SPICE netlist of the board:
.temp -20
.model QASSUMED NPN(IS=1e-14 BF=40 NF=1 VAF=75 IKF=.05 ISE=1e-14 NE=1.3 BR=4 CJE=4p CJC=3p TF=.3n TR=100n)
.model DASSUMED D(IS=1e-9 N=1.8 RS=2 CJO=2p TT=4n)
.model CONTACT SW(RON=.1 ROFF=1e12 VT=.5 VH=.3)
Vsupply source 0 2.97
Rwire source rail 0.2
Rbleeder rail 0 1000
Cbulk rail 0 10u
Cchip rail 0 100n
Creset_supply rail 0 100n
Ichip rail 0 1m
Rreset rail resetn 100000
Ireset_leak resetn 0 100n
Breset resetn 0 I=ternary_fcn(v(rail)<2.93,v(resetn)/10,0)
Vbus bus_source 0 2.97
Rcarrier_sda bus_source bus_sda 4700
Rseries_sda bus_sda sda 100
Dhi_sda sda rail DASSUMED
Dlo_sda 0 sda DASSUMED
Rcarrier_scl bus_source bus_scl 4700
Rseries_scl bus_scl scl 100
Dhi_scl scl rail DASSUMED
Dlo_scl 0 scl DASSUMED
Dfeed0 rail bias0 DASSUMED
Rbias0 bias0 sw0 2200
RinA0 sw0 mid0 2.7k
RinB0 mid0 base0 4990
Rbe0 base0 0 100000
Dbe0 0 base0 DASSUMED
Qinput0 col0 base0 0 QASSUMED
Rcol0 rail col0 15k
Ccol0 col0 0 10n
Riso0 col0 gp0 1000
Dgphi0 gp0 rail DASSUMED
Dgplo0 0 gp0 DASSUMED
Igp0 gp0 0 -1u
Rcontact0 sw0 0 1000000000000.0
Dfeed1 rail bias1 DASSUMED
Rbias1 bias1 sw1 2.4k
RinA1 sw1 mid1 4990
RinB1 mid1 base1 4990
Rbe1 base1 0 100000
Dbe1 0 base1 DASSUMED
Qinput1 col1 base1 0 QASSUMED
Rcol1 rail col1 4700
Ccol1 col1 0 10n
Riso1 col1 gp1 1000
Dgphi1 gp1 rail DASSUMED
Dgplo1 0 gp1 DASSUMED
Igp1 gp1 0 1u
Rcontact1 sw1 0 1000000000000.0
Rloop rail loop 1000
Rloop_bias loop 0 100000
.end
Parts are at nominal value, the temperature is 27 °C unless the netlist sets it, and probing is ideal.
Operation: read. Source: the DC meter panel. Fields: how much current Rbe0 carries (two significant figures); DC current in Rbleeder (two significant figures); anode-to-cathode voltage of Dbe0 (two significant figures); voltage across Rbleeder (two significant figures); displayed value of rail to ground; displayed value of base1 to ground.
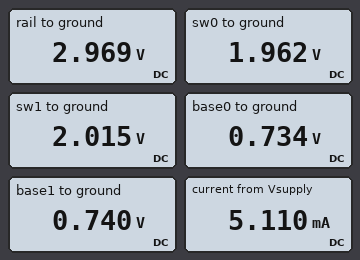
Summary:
7.3 µA
3.0 mA
-730 mV
3.0 V
2.969 V
0.740 V
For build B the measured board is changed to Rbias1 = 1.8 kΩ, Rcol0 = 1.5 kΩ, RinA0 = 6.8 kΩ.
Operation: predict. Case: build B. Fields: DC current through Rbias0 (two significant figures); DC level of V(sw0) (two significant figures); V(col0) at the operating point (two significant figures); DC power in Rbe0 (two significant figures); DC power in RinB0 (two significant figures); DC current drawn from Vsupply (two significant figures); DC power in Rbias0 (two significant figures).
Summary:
110 µA
2.1 V
56 mV
5.7 µW
63 µW
6.8 mA
28 µW
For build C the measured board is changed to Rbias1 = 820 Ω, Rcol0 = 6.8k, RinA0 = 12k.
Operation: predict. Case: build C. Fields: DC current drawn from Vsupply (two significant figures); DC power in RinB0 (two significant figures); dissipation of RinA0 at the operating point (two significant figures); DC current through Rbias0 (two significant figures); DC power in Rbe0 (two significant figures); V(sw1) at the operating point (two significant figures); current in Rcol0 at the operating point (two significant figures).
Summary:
5.3 mA
35 µW
84 µW
84 µA
5.3 µW
2.2 V
430 µA
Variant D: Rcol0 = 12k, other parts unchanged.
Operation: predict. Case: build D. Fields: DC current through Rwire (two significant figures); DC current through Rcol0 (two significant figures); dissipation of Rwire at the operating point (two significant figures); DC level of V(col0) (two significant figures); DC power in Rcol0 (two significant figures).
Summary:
5.2 mA
250 µA
5.3 µW
12 mV
730 µW
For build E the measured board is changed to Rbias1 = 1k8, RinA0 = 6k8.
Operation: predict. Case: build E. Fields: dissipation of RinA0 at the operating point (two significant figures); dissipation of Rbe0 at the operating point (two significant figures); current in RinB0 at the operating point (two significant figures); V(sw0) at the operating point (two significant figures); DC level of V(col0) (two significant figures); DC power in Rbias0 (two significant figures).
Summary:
89 µW
5.3 µW
110 µA
2.1 V
13 mV
29 µW
